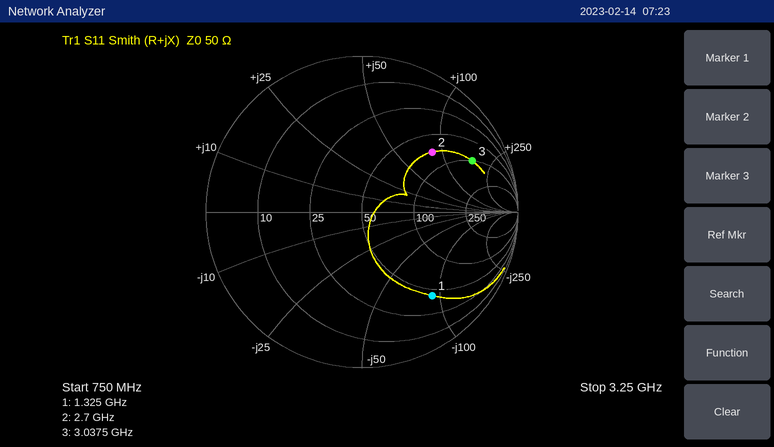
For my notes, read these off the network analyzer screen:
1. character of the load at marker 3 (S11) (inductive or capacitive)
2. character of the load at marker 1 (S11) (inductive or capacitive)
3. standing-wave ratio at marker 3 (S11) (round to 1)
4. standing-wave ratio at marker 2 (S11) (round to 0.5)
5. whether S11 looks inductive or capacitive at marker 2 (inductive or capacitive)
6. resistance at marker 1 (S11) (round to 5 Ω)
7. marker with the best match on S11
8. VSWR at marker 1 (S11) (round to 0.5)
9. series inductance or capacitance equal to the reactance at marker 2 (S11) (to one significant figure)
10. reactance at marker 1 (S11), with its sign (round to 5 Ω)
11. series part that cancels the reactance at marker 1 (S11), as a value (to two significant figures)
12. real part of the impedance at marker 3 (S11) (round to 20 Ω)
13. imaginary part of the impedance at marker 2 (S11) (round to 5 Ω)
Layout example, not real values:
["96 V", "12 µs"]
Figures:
["inductive", "capacitive", "8", "4.0", "inductive", "45 Ω", "marker 2", "5.5", "5 nH", "-90 Ω", "11 nH", "100 Ω", "+85 Ω"]
